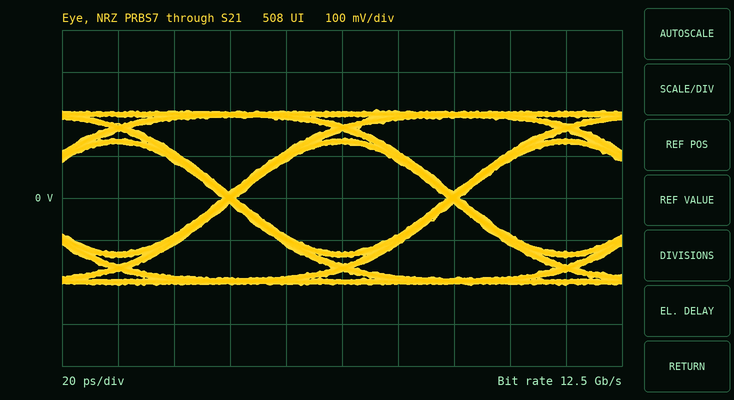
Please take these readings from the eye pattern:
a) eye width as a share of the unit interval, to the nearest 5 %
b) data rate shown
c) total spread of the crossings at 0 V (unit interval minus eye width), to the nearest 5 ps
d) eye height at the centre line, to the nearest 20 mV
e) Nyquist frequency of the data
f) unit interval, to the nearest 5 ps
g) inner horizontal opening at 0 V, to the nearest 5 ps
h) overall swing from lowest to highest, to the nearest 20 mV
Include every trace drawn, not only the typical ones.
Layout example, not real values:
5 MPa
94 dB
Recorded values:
95 %
12.5 Gb/s
5 ps
260 mV
6.25 GHz
80 ps
75 ps
420 mV
